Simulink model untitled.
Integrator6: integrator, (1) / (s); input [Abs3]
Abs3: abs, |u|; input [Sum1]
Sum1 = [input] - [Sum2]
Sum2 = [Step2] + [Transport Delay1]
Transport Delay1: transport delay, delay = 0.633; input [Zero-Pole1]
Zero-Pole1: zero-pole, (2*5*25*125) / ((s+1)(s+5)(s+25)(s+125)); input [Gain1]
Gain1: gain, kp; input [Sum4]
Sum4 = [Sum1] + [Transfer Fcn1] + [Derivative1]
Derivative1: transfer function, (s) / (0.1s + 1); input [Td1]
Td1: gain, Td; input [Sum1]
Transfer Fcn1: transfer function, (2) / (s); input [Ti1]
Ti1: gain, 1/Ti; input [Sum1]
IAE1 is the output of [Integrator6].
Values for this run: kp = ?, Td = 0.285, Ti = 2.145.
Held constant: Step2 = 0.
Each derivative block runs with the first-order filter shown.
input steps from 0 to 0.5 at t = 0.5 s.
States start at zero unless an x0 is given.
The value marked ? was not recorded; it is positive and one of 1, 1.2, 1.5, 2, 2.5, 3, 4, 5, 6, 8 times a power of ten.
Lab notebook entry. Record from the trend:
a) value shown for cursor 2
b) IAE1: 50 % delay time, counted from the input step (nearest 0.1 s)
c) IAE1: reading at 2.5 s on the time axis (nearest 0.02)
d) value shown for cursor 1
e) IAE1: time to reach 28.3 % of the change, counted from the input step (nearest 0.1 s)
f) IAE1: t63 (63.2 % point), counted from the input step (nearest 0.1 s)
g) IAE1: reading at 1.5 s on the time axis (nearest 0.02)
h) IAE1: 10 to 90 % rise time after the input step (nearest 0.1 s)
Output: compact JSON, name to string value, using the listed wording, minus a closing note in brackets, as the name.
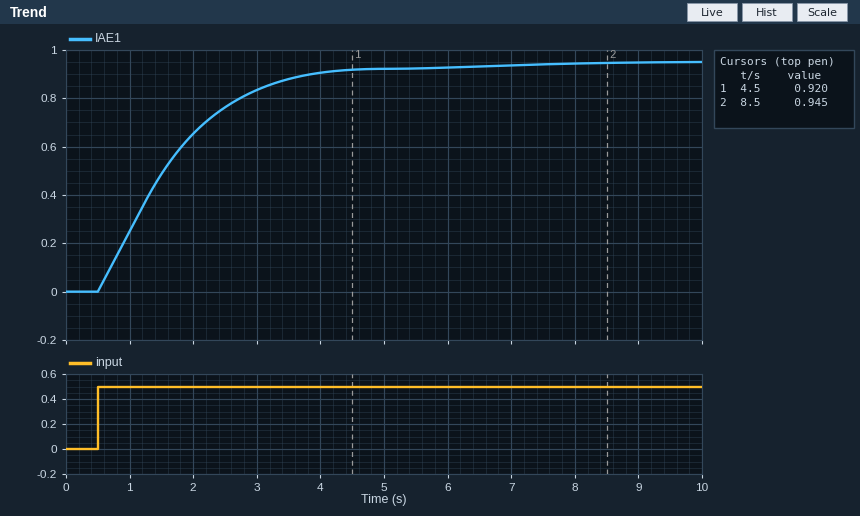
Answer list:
{"value shown for cursor 2": "0.945", "IAE1: 50 % delay time, counted from the input step": "1.0 s", "IAE1: reading at 2.5 s on the time axis": "0.76", "value shown for cursor 1": "0.920", "IAE1: time to reach 28.3 % of the change, counted from the input step": "0.5 s", "IAE1: t63 (63.2 % point), counted from the input step": "1.3 s", "IAE1: reading at 1.5 s on the time axis": "0.48", "IAE1: 10 to 90 % rise time after the input step": "2.5 s"}
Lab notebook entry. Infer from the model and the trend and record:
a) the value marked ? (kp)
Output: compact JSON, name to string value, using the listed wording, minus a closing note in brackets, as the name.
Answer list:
{"the value marked ?": "0.3"}
